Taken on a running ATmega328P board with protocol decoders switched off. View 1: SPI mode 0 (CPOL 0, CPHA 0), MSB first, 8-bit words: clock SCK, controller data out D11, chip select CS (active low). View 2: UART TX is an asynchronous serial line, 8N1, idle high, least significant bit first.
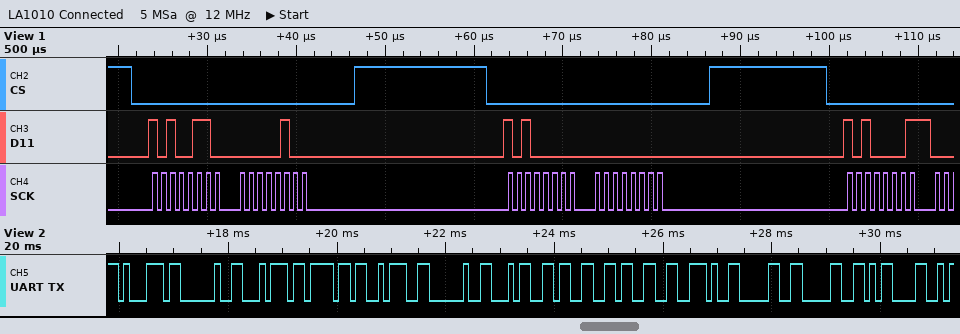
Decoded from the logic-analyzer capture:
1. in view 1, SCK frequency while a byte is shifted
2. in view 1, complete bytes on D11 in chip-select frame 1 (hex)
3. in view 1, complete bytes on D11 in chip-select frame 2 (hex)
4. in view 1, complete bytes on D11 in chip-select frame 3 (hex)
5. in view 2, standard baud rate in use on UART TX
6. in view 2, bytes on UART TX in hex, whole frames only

1 MHz
0xA6 0x04
0xA0 0x00
0xA1
9600 baud
0x71 0x20 0x74 0x6F 0x3A 0x20 0x34 0x33 0x33 0x2E 0x30 0x30 0x0D
